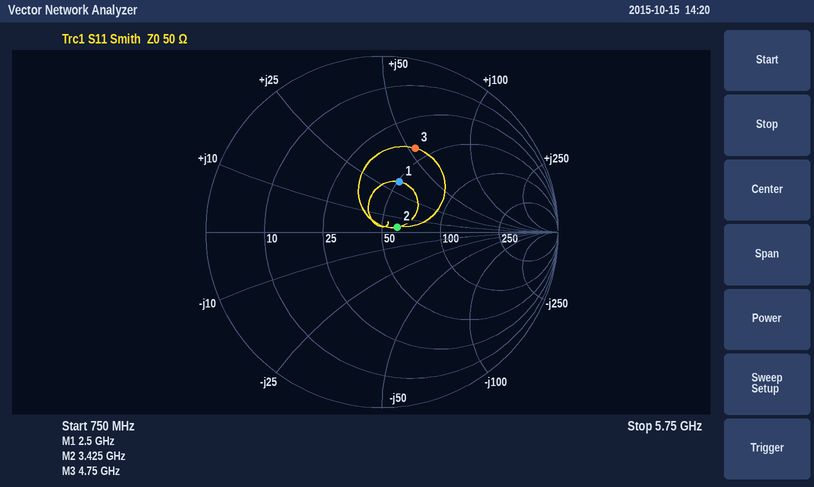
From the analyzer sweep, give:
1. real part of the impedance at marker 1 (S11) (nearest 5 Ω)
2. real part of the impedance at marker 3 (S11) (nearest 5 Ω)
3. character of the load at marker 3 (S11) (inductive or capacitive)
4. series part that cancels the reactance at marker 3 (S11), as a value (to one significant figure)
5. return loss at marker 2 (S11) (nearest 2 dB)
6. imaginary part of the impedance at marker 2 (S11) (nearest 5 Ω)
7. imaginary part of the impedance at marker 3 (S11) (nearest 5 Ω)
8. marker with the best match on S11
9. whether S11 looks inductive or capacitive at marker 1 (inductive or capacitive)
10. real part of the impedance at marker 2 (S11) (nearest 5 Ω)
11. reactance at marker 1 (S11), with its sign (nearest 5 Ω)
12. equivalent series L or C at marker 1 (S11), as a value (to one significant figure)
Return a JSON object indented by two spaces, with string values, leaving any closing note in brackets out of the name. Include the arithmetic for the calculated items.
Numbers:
{
  "real part of the impedance at marker 1 (S11)": "50 Ω",
  "real part of the impedance at marker 3 (S11)": "40 Ω",
  "character of the load at marker 3 (S11)": "inductive",
  "series part that cancels the reactance at marker 3 (S11), as a value": "C = 1/(2π × 4.75 GHz × 55 Ω) ≈ 609 fF, so 600 fF to one significant figure",
  "return loss at marker 2 (S11)": "20 dB",
  "imaginary part of the impedance at marker 2 (S11)": "+5 Ω",
  "imaginary part of the impedance at marker 3 (S11)": "+55 Ω",
  "marker with the best match on S11": "marker 2",
  "whether S11 looks inductive or capacitive at marker 1": "inductive",
  "real part of the impedance at marker 2 (S11)": "60 Ω",
  "reactance at marker 1 (S11), with its sign": "+30 Ω",
  "equivalent series L or C at marker 1 (S11), as a value": "L = 30 Ω/(2π × 2.5 GHz) ≈ 2 nH"
}
